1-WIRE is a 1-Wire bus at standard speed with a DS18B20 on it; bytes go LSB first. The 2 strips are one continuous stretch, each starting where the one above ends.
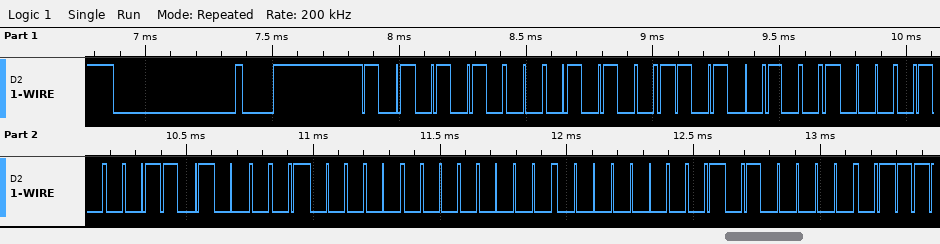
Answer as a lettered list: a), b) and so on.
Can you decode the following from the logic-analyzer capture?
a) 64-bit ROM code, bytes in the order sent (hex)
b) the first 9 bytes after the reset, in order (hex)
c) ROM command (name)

a) 28 4B 42 2C 04 00 00 05
b) 55 28 4B 42 2C 04 00 00 05
c) Match ROM
